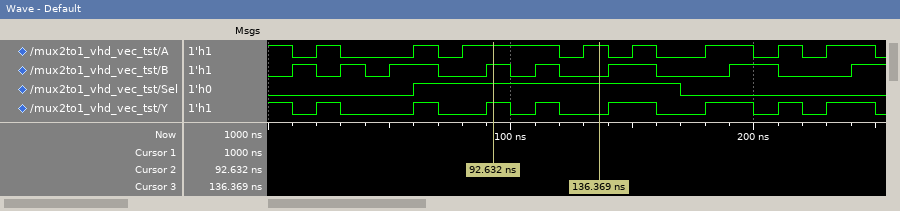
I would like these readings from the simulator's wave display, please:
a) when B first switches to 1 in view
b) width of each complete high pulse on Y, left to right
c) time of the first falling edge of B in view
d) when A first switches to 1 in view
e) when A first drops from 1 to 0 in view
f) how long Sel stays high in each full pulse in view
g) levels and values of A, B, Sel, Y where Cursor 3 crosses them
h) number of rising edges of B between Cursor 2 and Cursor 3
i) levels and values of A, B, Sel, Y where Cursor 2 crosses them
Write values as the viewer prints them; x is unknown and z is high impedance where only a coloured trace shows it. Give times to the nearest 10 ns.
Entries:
10 ns
10 ns, 10 ns, 10 ns, 10 ns, 20 ns, 20 ns, 10 ns, 20 ns
20 ns
20 ns
10 ns
110 ns
A=1, B=0, Sel=1, Y=0
1
A=1, B=1, Sel=1, Y=1
